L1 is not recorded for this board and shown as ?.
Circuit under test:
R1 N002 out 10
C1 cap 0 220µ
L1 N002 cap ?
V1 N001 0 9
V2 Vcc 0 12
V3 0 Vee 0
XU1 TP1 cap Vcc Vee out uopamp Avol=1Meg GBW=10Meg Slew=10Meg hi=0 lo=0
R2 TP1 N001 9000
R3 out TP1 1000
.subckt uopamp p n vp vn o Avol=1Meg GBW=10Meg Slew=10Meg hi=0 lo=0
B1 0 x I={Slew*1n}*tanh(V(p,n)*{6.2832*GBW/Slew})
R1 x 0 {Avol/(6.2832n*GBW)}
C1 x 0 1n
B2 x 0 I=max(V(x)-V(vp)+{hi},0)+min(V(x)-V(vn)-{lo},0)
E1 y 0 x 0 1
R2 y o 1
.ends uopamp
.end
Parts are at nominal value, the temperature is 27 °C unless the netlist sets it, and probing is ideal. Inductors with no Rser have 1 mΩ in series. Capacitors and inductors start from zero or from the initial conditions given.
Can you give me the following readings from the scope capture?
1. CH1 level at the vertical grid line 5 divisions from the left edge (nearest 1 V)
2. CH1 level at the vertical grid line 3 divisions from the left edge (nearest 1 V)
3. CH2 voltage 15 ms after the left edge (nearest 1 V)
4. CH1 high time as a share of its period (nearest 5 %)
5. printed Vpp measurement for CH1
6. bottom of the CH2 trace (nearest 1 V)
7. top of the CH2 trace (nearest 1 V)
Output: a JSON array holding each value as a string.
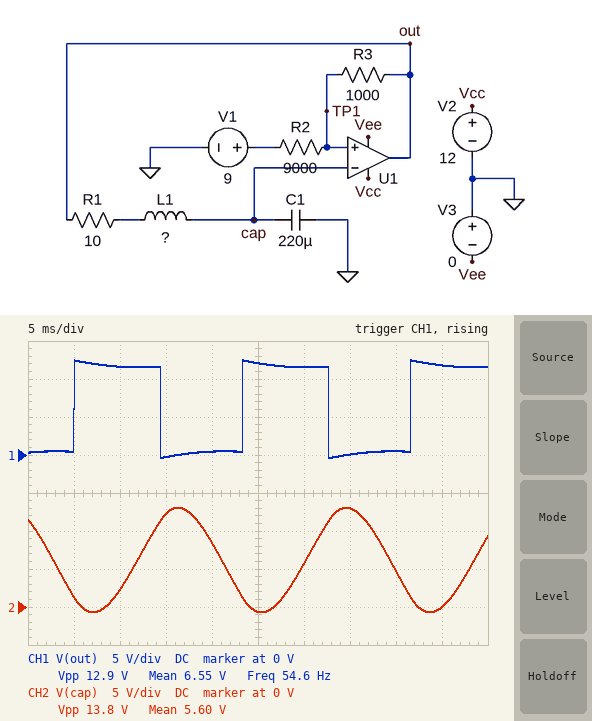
["12 V", "0 V", "12 V", "50 %", "12.9 V", "-1 V", "13 V"]
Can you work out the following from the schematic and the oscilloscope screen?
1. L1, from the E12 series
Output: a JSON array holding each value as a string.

["68 mH"]
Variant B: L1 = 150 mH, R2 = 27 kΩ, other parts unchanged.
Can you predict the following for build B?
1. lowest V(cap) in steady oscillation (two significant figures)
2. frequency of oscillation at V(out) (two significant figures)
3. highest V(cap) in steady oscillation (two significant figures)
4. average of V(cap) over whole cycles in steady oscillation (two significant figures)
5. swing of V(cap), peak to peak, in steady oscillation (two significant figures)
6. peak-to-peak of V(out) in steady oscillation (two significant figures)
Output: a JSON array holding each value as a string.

["-2.7 V", "36 Hz", "15 V", "6.0 V", "17 V", "13 V"]
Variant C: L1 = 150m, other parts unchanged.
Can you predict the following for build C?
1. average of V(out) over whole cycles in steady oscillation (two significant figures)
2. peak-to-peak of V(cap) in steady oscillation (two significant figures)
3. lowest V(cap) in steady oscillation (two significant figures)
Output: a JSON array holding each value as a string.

["6.1 V", "17 V", "-2.2 V"]
